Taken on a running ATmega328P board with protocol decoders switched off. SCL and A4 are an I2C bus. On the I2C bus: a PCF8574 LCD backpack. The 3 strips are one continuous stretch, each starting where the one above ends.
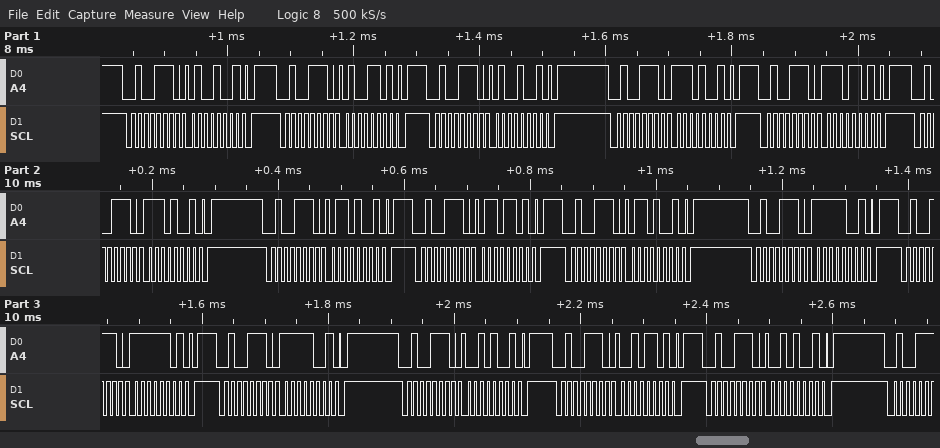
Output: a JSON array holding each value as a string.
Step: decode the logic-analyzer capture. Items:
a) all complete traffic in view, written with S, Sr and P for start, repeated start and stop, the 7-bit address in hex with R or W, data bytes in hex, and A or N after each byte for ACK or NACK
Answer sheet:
["S 27W A 49 A P S 27W A 4D A P S 27W A 49 A P S 27W A E9 A P S 27W A ED A P S 27W A E9 A P S 27W A 69 A P S 27W A 6D A P S 27W A 69 A P S 27W A F9 A P S 27W A FD A P S 27W A F9 A P S 27W A 29 A P S 27W A 2D A P S 27W A 29 A P"]
